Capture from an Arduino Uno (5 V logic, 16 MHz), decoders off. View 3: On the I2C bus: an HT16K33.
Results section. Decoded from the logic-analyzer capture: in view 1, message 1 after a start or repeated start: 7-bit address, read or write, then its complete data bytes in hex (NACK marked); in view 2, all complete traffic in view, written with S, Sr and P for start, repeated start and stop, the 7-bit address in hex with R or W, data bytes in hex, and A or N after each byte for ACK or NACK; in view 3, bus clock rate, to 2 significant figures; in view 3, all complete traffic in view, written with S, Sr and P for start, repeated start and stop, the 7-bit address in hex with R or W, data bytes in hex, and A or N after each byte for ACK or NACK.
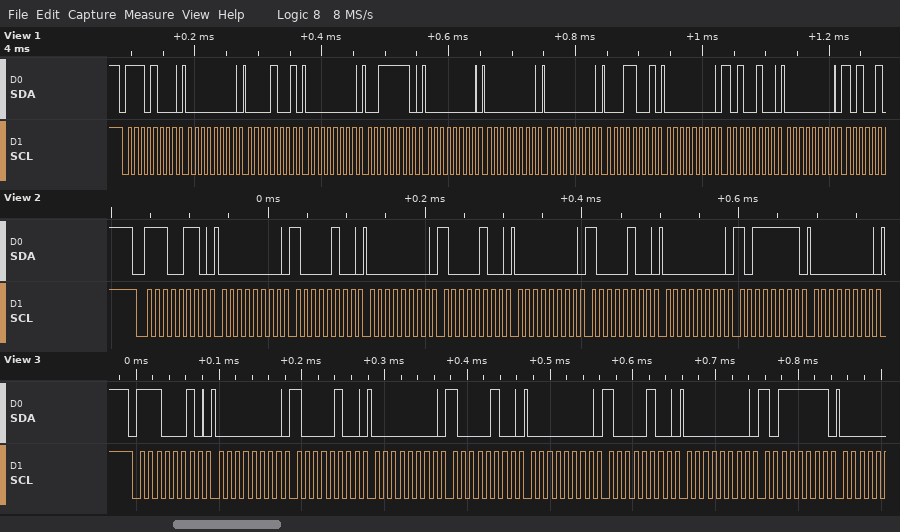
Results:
0x74 write: 00 09 00 3E 00 00 00 19 00 A4 00
S 73W A 00 A 84 A 00 A 84 A 00 A 84 A 00 A BF A 00 A
100 kHz
S 71W A 00 A 84 A 00 A 84 A 00 A 84 A 00 A BF A
